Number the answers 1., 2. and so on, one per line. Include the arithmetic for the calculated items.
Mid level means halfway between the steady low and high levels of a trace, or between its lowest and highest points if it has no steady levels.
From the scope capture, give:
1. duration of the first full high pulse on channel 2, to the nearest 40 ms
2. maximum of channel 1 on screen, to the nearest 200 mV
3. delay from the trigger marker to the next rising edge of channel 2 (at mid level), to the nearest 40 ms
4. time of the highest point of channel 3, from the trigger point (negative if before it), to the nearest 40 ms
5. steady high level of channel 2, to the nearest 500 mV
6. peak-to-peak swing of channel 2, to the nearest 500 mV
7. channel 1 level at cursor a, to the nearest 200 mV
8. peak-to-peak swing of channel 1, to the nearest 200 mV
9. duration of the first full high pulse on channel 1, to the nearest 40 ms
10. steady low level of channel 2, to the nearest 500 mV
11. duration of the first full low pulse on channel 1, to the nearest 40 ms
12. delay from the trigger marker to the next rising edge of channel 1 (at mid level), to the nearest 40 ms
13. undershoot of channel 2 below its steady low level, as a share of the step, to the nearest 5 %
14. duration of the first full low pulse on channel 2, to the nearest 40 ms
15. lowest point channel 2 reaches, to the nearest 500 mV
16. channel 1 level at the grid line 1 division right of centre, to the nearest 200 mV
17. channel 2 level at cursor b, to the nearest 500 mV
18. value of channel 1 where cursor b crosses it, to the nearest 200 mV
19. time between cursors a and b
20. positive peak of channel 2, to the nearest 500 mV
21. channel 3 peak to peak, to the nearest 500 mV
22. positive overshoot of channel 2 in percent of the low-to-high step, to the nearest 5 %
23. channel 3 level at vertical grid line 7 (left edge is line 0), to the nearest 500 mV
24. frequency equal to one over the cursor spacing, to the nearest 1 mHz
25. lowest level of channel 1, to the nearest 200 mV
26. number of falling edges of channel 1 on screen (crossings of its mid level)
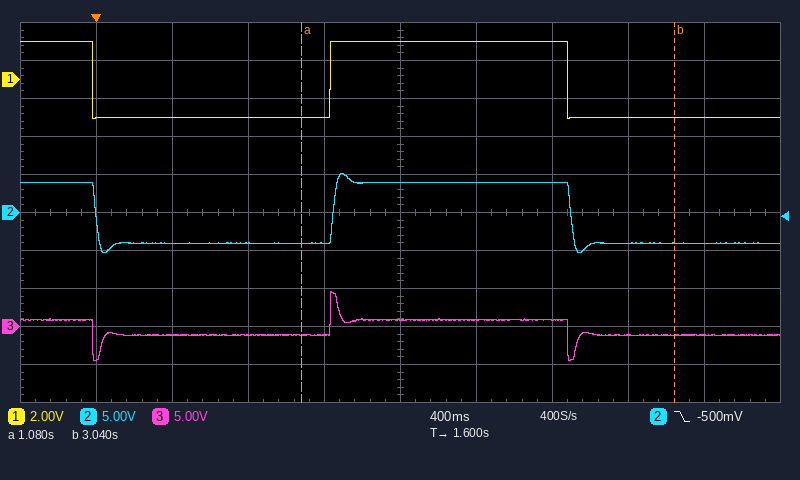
1. 1.24 s
2. 2.0 V
3. 1.24 s
4. +1.24 s
5. 4.0 V
6. 5.0 V − (-5.5 V) = 10.5 V
7. -2.0 V
8. 2.0 V − (-2.0 V) = 4.0 V
9. 1.24 s
10. -4.0 V
11. 1.24 s
12. 1.24 s
13. 15 %
14. 1.24 s
15. -5.5 V
16. 2.0 V
17. -4.0 V
18. -2.0 V
19. 3.04 s − (1.08 s) = 1.96 s
20. 5.0 V
21. 4.5 V − (-4.5 V) = 9.0 V
22. 15 %
23. 1.0 V
24. 1 / 1.96 s ≈ 510 mHz
25. -2.0 V
26. 2
